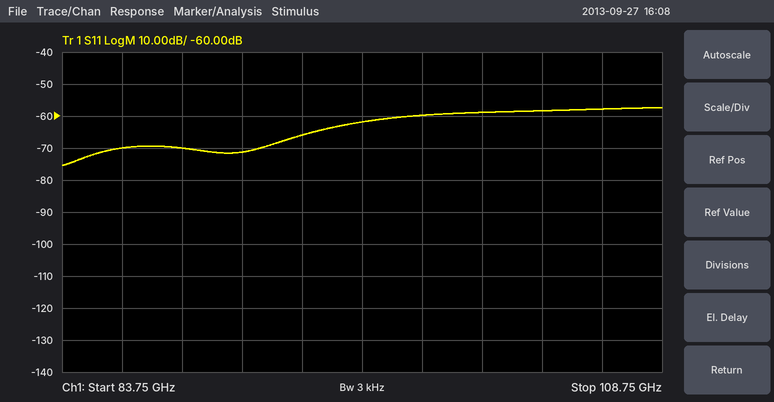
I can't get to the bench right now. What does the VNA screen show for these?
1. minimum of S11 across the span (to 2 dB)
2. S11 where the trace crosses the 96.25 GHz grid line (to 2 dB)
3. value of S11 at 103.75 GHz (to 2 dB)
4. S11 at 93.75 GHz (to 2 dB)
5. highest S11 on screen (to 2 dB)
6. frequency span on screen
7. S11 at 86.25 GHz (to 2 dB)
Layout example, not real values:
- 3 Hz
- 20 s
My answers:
- -76 dB
- -62 dB
- -58 dB
- -66 dB
- -58 dB
- 25 GHz
- -70 dB
